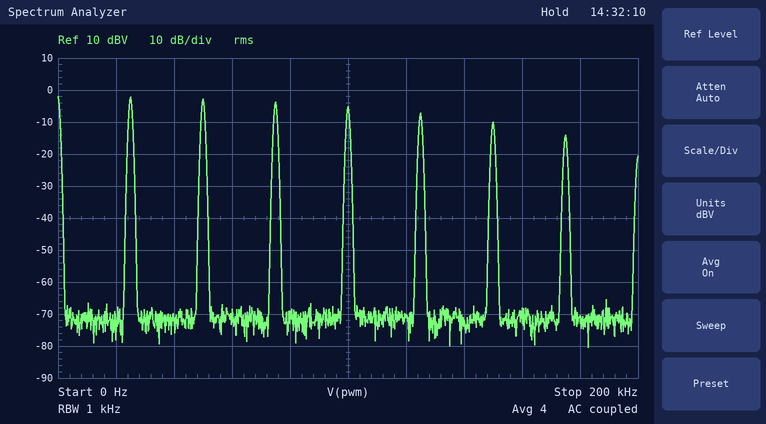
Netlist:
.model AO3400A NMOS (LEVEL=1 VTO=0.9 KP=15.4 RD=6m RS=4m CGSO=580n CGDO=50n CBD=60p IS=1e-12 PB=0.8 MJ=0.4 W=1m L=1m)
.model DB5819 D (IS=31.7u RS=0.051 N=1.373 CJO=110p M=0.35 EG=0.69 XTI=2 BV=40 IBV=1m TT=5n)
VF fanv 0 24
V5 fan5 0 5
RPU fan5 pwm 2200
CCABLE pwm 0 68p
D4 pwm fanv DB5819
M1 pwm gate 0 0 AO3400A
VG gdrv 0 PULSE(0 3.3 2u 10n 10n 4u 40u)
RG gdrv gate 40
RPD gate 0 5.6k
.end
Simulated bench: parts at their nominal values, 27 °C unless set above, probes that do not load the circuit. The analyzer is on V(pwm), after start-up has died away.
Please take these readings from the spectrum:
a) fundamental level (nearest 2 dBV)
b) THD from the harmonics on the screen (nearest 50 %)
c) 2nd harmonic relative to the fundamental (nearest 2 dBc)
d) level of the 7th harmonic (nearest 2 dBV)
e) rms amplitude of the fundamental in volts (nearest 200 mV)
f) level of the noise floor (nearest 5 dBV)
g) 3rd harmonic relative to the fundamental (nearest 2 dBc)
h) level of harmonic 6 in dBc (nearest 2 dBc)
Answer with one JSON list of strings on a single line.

["-2 dBV", "150 %", "0 dBc", "-14 dBV", "800 mV", "-70 dBV", "-2 dBc", "-8 dBc"]
